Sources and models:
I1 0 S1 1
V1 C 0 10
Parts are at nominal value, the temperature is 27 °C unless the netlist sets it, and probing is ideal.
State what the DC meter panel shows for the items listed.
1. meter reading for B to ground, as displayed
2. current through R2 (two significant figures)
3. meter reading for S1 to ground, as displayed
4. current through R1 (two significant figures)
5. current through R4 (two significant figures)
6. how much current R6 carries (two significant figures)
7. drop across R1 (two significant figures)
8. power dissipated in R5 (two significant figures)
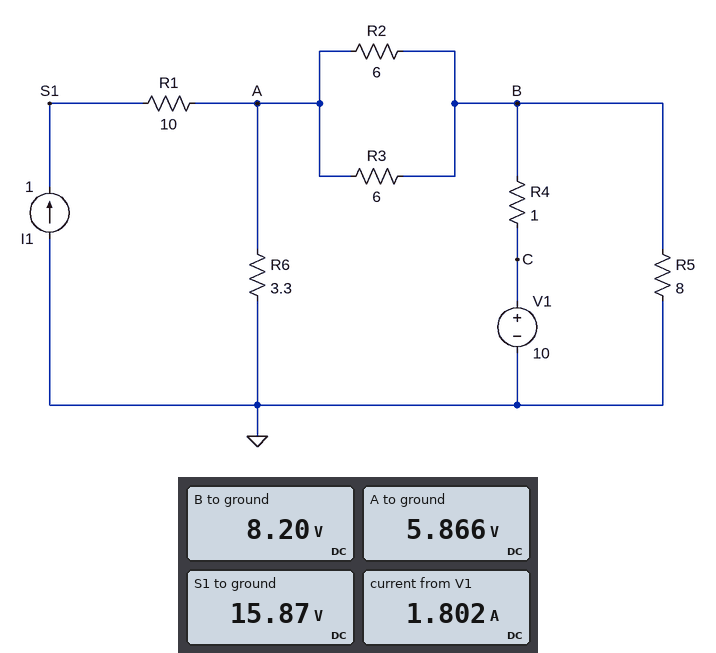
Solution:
8.20 V
390 mA
15.87 V
1.0 A
1.8 A
1.8 A
10 V
8.4 W
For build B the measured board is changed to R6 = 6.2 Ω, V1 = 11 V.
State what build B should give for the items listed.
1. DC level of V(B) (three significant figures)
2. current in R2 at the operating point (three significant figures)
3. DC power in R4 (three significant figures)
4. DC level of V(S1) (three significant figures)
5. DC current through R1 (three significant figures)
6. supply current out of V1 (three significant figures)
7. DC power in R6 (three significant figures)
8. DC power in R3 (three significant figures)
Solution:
9.46 V
177 mA
2.36 W
18.4 V
1.00 A
1.54 A
11.4 W
189 mW
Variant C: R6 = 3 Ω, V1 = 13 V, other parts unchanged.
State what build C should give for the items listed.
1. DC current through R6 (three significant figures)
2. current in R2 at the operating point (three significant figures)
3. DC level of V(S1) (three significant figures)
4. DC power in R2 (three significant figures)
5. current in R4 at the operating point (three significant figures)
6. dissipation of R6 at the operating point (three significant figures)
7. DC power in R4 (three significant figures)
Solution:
2.24 A
621 mA
16.7 V
2.31 W
2.55 A
15.1 W
6.49 W
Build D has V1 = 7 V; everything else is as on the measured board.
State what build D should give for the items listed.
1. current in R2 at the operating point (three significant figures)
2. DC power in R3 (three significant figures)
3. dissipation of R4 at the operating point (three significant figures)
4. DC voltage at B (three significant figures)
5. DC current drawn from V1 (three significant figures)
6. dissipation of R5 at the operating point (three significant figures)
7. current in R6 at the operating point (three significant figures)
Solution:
203 mA
248 mW
1.30 W
5.86 V
1.14 A
4.29 W
1.41 A
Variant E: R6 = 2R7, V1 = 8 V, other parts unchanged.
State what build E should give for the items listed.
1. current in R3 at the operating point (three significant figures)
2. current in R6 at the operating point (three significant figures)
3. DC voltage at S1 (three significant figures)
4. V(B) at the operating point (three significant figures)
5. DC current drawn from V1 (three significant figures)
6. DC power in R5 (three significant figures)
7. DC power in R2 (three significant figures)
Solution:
335 mA
1.67 A
14.5 V
6.52 V
1.48 A
5.31 W
672 mW
